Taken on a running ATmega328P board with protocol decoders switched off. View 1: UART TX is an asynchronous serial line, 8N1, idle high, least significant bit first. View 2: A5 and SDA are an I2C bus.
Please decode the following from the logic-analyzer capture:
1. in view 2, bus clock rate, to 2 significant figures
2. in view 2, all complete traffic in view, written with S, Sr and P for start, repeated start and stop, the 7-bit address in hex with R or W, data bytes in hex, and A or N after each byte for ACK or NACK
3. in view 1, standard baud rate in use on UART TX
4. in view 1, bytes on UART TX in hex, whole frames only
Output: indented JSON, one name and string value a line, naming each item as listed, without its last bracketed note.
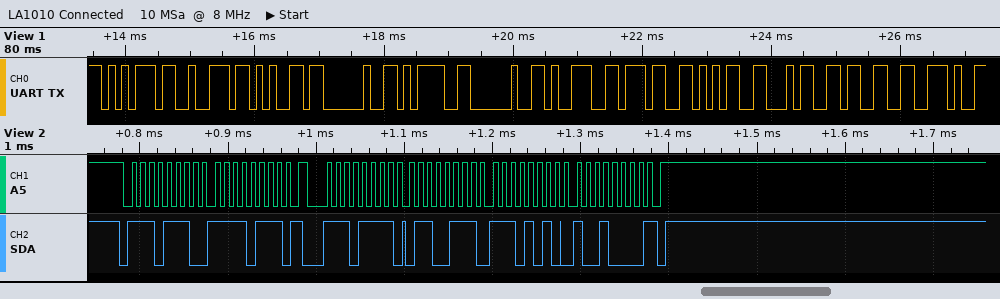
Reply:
{
  "in view 2, bus clock rate, to 2 significant figures": "100 kHz",
  "in view 2, all complete traffic in view, written with S, Sr and P for start, repeated start and stop, the 7-bit address in hex with R or W, data bytes in hex, and A or N after each byte for ACK or NACK": "S 77W A F7 A Sr 77R A 67 A EA A 90 N P",
  "in view 1, standard baud rate in use on UART TX": "9600 baud",
  "in view 1, bytes on UART TX in hex, whole frames only": "0x75 0x72 0x65 0x20 0x3D 0x20 0x39 0x37 0x35 0x34 0x33 0x2E"
}
